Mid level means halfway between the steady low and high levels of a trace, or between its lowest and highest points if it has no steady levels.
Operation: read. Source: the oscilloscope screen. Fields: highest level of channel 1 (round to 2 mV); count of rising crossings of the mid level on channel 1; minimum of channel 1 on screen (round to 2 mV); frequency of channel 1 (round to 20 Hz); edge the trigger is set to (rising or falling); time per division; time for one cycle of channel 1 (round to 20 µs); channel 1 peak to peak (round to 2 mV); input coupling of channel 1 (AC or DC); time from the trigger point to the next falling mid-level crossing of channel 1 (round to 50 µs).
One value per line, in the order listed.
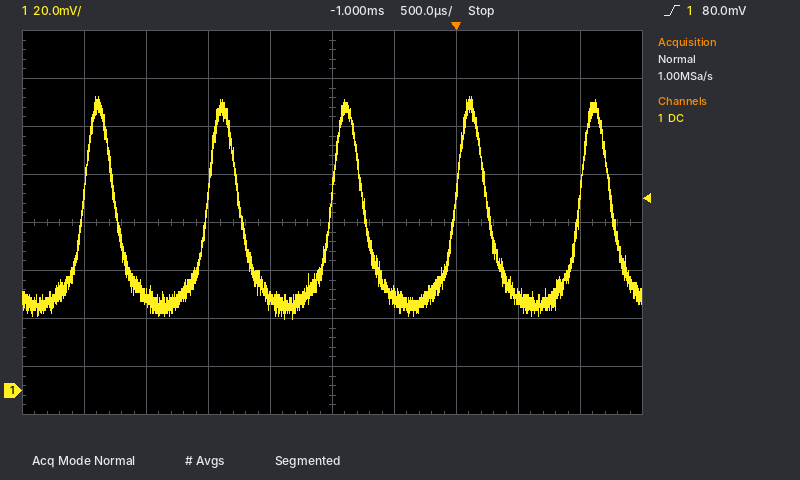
122 mV
5
30 mV
1.00 kHz
rising
500 µs
1.00 ms
92 mV
DC
250 µs
